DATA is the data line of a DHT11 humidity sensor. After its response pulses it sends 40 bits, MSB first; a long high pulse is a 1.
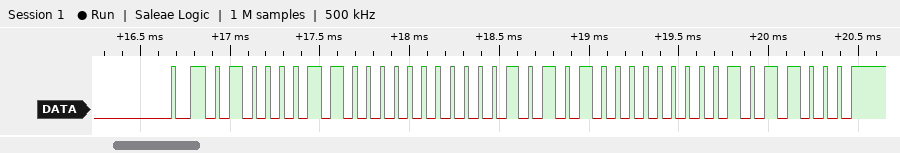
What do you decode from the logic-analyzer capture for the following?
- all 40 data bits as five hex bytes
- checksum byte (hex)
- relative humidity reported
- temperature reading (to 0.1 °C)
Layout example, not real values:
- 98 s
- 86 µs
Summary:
- 43 00 15 00 58
- 0x58
- 67 %
- 21.0 °C
